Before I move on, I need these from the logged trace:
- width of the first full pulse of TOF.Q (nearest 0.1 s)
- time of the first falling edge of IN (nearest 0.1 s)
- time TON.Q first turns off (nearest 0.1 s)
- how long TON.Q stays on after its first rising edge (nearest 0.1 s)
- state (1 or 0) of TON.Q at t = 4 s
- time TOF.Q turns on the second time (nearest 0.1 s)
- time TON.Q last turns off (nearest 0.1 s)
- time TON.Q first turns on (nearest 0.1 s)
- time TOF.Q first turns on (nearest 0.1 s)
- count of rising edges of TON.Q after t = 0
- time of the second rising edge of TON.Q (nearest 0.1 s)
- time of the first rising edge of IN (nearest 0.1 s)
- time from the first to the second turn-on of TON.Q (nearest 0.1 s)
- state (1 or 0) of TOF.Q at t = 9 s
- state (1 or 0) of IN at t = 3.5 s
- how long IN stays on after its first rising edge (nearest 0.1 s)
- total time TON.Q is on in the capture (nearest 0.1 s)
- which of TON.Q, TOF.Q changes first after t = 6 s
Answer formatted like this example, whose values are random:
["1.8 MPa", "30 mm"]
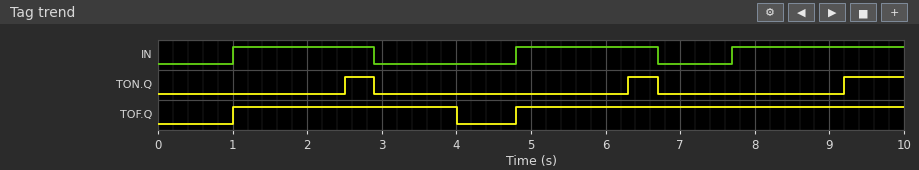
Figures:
["3.0 s", "2.9 s", "2.9 s", "0.4 s", "0", "4.8 s", "6.7 s", "2.5 s", "1.0 s", "3", "6.3 s", "1.0 s", "3.8 s", "1", "0", "1.9 s", "1.6 s", "TON.Q"]
